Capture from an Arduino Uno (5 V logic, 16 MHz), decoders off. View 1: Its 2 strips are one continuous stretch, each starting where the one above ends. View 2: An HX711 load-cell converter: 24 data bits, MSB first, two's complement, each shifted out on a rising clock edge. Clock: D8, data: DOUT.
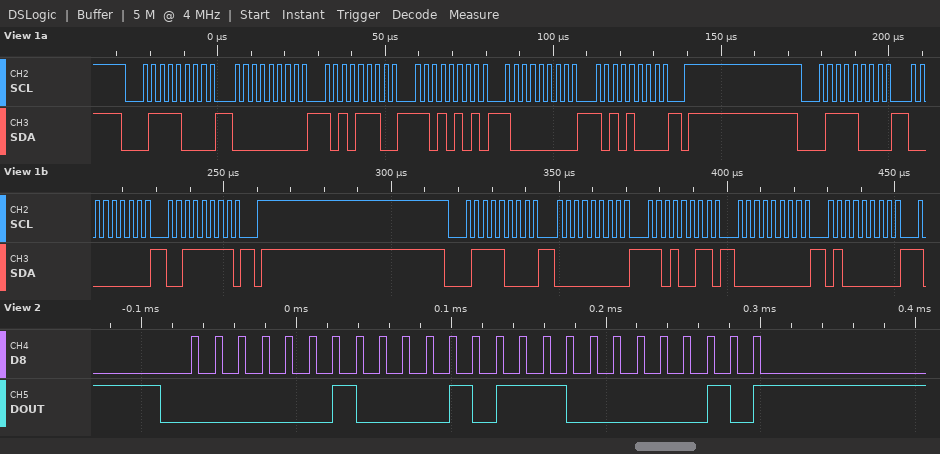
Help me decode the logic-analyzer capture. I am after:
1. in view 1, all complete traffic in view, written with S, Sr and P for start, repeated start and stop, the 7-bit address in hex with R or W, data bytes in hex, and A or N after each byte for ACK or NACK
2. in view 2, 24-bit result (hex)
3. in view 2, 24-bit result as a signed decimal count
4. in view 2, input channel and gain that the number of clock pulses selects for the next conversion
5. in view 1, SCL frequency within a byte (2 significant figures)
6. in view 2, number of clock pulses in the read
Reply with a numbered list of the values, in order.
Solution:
1. S 3CW A 00 A AE A D5 A 80 A A8 A P S 3CW A 00 A 3F A P S 3CW A 00 A D3 A 00 A 40 A
2. 0x021702
3. 136962
4. channel A, gain 128
5. 400 kHz
6. 25
